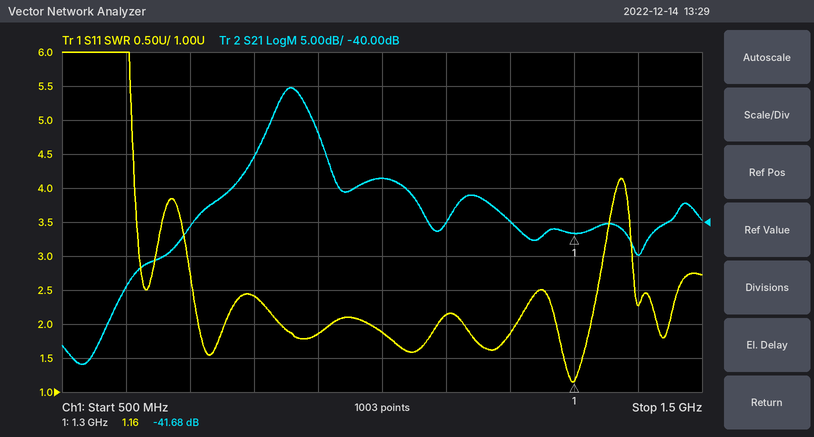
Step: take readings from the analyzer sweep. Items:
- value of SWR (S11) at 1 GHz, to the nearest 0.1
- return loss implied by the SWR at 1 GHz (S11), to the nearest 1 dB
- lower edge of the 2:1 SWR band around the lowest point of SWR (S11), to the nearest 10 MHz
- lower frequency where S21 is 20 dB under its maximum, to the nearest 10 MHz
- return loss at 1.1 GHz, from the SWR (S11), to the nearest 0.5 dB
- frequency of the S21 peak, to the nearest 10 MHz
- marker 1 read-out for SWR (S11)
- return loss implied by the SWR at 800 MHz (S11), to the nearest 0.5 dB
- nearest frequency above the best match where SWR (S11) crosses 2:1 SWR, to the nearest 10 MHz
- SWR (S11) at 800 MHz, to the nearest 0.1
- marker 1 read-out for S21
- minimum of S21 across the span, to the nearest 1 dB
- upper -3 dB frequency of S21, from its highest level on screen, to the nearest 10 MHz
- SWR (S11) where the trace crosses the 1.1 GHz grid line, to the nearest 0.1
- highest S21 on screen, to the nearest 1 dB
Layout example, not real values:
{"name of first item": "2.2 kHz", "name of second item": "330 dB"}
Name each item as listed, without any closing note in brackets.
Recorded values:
{"value of SWR (S11) at 1 GHz, to the nearest 0.1": "1.9", "return loss implied by the SWR at 1 GHz (S11), to the nearest 1 dB": "10 dB", "lower edge of the 2:1 SWR band around the lowest point of SWR (S11), to the nearest 10 MHz": "1.27 GHz", "lower frequency where S21 is 20 dB under its maximum, to the nearest 10 MHz": "700 MHz", "return loss at 1.1 GHz, from the SWR (S11), to the nearest 0.5 dB": "9.0 dB", "frequency of the S21 peak, to the nearest 10 MHz": "860 MHz", "marker 1 read-out for SWR": "1.16", "return loss implied by the SWR at 800 MHz (S11), to the nearest 0.5 dB": "7.5 dB", "nearest frequency above the best match where SWR (S11) crosses 2:1 SWR, to the nearest 10 MHz": "1.33 GHz", "SWR (S11) at 800 MHz, to the nearest 0.1": "2.4", "marker 1 read-out for S21": "-41.68 dB", "minimum of S21 across the span, to the nearest 1 dB": "-61 dB", "upper -3 dB frequency of S21, from its highest level on screen, to the nearest 10 MHz": "880 MHz", "SWR (S11) where the trace crosses the 1.1 GHz grid line, to the nearest 0.1": "2.1", "highest S21 on screen, to the nearest 1 dB": "-20 dB"}
